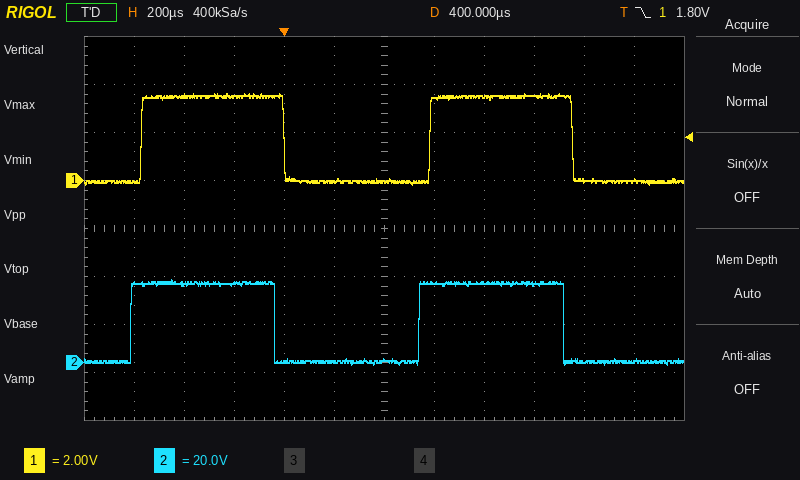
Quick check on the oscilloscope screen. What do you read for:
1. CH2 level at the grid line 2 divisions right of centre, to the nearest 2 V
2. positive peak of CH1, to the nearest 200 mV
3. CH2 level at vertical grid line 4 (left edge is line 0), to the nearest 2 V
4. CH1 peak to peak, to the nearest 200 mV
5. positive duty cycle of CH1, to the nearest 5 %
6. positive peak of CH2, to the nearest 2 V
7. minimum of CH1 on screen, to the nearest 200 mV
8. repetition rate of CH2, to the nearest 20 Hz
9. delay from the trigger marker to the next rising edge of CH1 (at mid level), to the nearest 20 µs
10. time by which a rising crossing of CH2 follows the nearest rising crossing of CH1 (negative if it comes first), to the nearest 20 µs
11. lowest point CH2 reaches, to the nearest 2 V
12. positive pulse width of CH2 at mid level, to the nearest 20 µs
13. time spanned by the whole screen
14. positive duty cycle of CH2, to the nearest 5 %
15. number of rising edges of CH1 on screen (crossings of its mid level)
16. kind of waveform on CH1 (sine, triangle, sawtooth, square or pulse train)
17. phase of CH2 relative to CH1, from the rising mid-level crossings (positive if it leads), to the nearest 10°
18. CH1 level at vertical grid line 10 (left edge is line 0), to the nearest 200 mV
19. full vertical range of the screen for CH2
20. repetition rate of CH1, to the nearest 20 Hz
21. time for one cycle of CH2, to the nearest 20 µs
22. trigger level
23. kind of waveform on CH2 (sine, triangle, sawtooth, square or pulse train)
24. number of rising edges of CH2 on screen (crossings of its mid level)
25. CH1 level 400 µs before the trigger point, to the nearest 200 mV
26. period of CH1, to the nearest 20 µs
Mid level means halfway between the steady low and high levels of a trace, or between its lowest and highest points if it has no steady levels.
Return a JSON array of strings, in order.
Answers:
["34 V", "3.6 V", "0 V", "3.8 V", "50 %", "34 V", "-200 mV", "860 Hz", "580 µs", "-40 µs", "0 V", "580 µs", "2.4 ms", "50 %", "2", "square", "+10°", "0.0 V", "160 V", "860 Hz", "1.16 ms", "1.80 V", "square", "2", "3.6 V", "1.16 ms"]
